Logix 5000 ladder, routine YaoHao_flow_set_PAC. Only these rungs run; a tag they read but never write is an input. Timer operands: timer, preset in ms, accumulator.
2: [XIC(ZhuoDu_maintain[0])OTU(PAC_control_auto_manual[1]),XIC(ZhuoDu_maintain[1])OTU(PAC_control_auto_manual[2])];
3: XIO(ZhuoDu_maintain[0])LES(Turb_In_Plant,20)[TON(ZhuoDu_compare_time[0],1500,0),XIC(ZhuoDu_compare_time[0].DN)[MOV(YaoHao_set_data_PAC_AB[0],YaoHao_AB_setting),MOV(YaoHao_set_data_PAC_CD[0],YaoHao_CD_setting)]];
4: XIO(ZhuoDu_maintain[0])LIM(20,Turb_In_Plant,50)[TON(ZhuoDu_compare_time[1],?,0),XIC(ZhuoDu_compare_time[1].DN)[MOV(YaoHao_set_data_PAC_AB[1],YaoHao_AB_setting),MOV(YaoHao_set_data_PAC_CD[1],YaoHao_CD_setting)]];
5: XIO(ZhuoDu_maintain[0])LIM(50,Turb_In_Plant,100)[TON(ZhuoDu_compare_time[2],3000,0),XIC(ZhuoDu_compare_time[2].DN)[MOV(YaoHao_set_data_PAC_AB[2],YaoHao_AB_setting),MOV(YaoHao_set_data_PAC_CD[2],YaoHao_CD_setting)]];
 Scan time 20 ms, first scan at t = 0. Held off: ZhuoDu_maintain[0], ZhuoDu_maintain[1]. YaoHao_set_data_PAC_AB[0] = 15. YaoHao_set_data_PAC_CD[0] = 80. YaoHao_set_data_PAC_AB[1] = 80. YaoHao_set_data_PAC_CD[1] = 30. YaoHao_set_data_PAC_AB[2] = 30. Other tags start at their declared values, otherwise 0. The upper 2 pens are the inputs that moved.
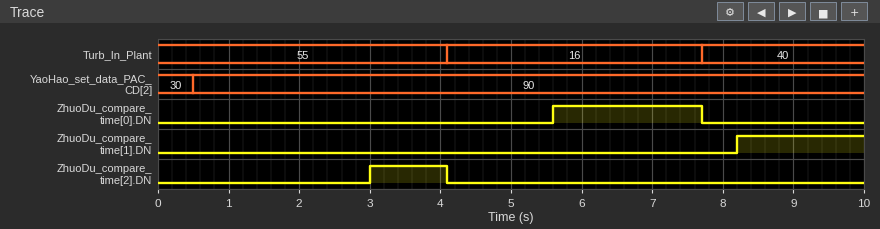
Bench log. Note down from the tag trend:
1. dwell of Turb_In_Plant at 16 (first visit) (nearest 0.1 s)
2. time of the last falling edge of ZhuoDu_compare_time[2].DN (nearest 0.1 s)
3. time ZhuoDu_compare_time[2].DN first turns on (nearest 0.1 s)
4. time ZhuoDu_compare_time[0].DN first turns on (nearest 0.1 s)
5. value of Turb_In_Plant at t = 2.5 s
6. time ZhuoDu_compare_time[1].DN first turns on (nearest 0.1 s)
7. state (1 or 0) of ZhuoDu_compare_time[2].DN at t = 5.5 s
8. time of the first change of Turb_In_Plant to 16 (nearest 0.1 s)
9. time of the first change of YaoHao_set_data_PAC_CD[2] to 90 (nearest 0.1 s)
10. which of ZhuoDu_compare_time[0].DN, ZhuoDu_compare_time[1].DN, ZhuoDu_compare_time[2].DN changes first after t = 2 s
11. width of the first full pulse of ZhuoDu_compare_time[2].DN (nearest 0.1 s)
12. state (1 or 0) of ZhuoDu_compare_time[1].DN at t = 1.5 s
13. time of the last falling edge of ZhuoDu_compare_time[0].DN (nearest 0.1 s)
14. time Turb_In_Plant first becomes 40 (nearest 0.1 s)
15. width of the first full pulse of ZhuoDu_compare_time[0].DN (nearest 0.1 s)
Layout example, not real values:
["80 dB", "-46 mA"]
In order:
["3.6 s", "4.1 s", "3.0 s", "5.6 s", "55", "8.2 s", "0", "4.1 s", "0.5 s", "ZhuoDu_compare_time[2].DN", "1.1 s", "0", "7.7 s", "7.7 s", "2.1 s"]
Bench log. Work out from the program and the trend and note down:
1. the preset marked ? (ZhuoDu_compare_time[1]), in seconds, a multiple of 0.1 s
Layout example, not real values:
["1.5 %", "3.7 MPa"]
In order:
["0.5 s"]
